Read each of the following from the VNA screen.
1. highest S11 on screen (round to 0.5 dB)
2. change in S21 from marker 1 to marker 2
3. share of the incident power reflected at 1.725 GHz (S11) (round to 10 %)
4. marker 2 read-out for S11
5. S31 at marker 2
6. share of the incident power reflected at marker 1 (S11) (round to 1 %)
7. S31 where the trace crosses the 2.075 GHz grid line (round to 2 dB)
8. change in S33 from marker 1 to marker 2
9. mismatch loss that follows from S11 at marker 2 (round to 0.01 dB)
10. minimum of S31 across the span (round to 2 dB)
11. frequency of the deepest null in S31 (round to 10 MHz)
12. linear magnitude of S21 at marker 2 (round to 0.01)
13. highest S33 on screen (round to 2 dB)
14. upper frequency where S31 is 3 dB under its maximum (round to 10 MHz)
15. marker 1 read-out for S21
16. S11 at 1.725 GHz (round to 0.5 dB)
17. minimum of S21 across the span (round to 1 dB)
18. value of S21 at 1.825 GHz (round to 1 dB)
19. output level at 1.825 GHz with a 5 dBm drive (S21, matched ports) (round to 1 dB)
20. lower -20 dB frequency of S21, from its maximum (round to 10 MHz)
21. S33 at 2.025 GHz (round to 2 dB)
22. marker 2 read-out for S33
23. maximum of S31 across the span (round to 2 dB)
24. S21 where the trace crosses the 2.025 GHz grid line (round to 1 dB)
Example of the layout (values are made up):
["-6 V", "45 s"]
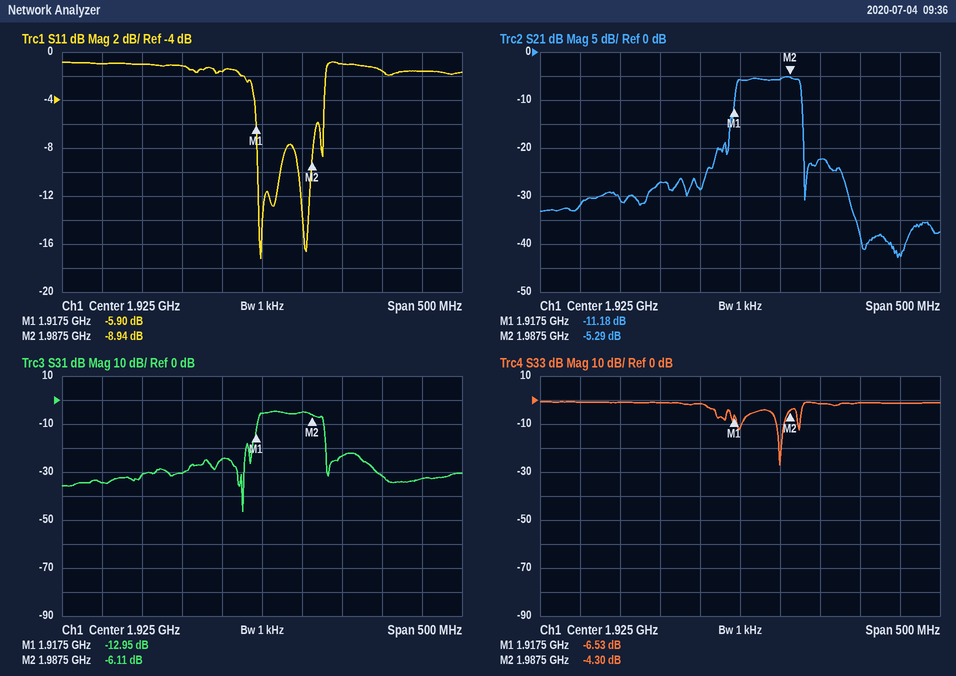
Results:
["-1.0 dB", "5.89 dB", "80 %", "-8.94 dB", "-6.11 dB", "26 %", "-32 dB", "2.23 dB", "0.59 dB", "-46 dB", "1.90 GHz", "0.54", "0 dB", "2.00 GHz", "-11.18 dB", "-1.0 dB", "-43 dB", "-27 dB", "-22 dBm", "1.88 GHz", "-2 dB", "-4.30 dB", "-4 dB", "-22 dB"]
